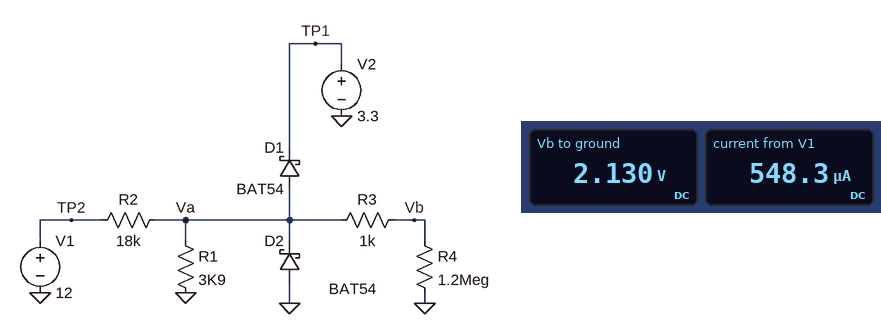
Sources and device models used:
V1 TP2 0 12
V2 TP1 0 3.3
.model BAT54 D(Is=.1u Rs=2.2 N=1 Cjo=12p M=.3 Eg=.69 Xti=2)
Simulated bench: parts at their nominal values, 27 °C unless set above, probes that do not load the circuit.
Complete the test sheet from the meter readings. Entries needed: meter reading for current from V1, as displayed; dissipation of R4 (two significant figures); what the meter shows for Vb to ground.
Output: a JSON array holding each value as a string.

["548.3 µA", "3.8 µW", "2.130 V"]
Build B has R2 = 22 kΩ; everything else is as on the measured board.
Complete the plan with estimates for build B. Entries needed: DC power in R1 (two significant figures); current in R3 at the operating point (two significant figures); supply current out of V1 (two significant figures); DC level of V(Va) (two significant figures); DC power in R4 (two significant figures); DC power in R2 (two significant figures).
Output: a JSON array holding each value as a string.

["830 µW", "1.5 µA", "460 µA", "1.8 V", "2.7 µW", "4.7 mW"]
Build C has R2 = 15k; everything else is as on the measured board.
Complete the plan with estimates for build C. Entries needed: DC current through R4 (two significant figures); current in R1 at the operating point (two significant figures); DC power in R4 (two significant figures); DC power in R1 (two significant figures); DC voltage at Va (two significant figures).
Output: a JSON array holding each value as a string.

["2.1 µA", "630 µA", "5.1 µW", "1.6 mW", "2.5 V"]
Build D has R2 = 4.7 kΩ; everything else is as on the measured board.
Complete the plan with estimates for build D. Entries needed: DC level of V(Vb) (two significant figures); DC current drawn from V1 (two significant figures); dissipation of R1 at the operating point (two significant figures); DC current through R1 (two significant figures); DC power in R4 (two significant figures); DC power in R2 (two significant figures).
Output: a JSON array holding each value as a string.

["3.5 V", "1.8 mA", "3.2 mW", "910 µA", "10 µW", "15 mW"]
